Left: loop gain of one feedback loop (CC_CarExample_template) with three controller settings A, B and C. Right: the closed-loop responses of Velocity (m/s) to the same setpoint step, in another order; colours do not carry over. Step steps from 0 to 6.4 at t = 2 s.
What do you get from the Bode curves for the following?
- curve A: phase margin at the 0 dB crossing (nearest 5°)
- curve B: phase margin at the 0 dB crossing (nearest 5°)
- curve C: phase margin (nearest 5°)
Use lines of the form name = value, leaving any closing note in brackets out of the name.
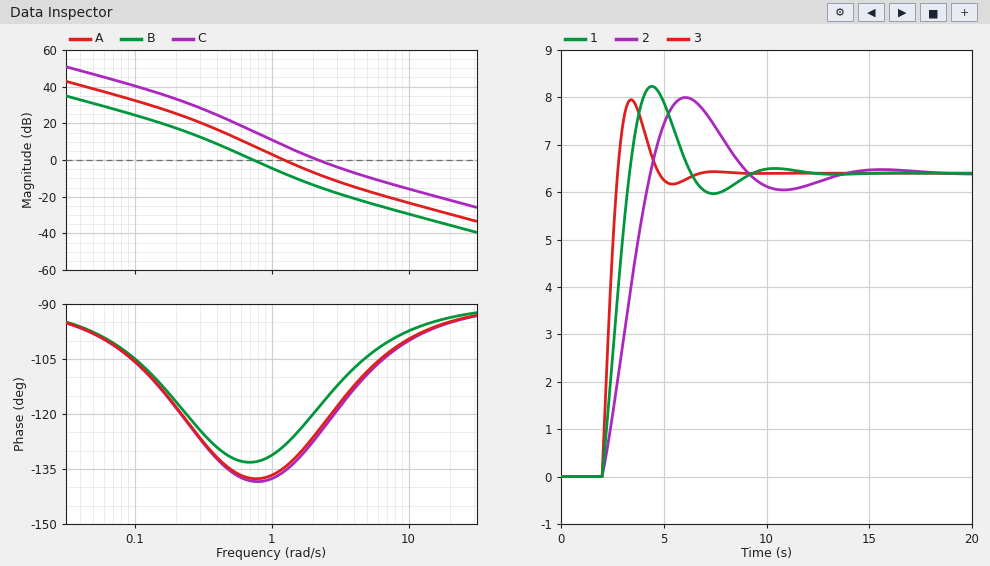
curve A: phase margin at the 0 dB crossing = 45°
curve B: phase margin at the 0 dB crossing = 45°
curve C: phase margin = 55°
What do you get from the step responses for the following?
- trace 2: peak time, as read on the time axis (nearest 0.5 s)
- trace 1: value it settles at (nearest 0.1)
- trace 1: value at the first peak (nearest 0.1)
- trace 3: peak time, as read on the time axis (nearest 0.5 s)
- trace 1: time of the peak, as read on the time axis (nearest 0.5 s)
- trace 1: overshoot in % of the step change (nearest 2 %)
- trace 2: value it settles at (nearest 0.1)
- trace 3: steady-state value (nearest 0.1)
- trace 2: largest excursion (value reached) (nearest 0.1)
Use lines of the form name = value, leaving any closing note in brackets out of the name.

trace 2: peak time, as read on the time axis = 6.0 s
trace 1: value it settles at = 6.4
trace 1: value at the first peak = 8.2
trace 3: peak time, as read on the time axis = 3.5 s
trace 1: time of the peak, as read on the time axis = 4.5 s
trace 1: overshoot in % of the step change = 28 %
trace 2: value it settles at = 6.4
trace 3: steady-state value = 6.4
trace 2: largest excursion (value reached) = 8.0
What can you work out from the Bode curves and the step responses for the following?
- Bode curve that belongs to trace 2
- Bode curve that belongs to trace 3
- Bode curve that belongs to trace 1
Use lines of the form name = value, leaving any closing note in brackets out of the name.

Bode curve that belongs to trace 2 = B
Bode curve that belongs to trace 3 = C
Bode curve that belongs to trace 1 = A
